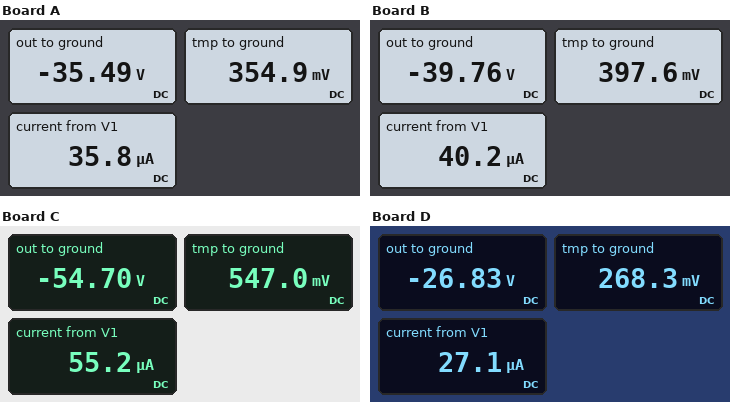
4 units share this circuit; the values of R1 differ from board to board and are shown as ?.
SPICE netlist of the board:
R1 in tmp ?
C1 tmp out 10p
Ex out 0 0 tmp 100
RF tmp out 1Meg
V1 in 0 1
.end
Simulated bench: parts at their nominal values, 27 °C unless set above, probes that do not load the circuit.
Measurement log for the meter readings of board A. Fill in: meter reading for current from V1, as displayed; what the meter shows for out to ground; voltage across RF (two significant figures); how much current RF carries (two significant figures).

35.8 µA
-35.49 V
36 V
36 µA
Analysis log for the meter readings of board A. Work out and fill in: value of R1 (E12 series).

18 kΩ
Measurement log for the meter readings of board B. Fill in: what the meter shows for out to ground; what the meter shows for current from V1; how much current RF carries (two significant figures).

-39.76 V
40.2 µA
40 µA
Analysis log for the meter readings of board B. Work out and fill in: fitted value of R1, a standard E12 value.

15 kΩ
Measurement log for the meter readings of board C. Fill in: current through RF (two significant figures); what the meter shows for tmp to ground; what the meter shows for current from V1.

55 µA
547.0 mV
55.2 µA
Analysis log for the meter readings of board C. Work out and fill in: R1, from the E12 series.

8.2 kΩ
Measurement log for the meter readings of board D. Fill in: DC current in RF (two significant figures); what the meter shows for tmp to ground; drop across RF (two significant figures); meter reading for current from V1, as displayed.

27 µA
268.3 mV
27 V
27.1 µA
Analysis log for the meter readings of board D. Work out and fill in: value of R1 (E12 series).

27 kΩ
